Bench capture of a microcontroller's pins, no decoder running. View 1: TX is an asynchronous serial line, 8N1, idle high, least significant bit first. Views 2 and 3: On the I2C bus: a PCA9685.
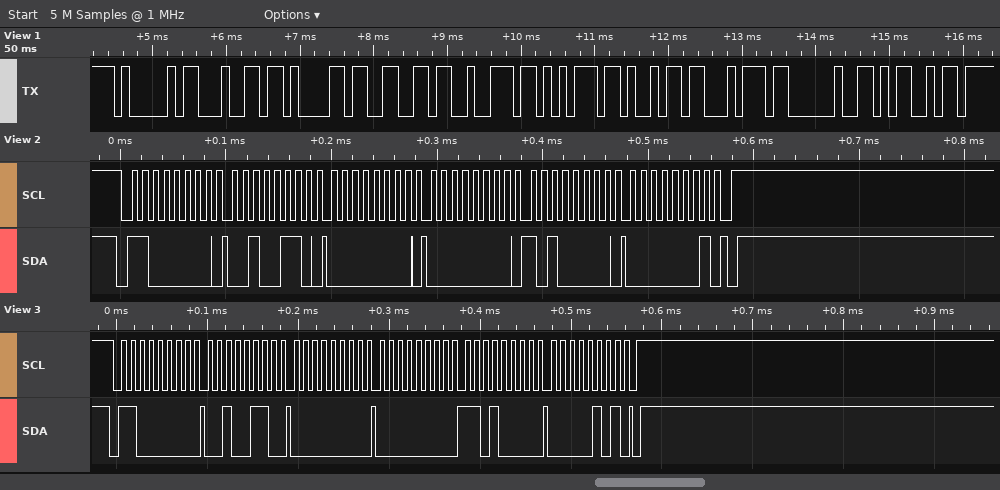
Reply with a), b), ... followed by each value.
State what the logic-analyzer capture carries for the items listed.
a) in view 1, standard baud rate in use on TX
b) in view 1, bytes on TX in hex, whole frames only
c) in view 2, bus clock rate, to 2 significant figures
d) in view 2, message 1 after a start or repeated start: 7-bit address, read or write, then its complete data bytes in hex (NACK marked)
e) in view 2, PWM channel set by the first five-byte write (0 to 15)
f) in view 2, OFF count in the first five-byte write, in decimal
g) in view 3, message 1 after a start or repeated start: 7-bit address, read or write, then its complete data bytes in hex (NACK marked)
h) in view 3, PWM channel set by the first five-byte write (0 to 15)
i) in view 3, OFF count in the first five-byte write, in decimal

a) 9600 baud
b) 0x41 0x64 0x61 0x66 0x72 0x75 0x69 0x74 0x20 0x4D
c) 100 kHz
d) 0x60 write: 26 00 00 A0 01
e) 8
f) 416
g) 0x60 write: 26 00 00 D0 05
h) 8
i) 1488
